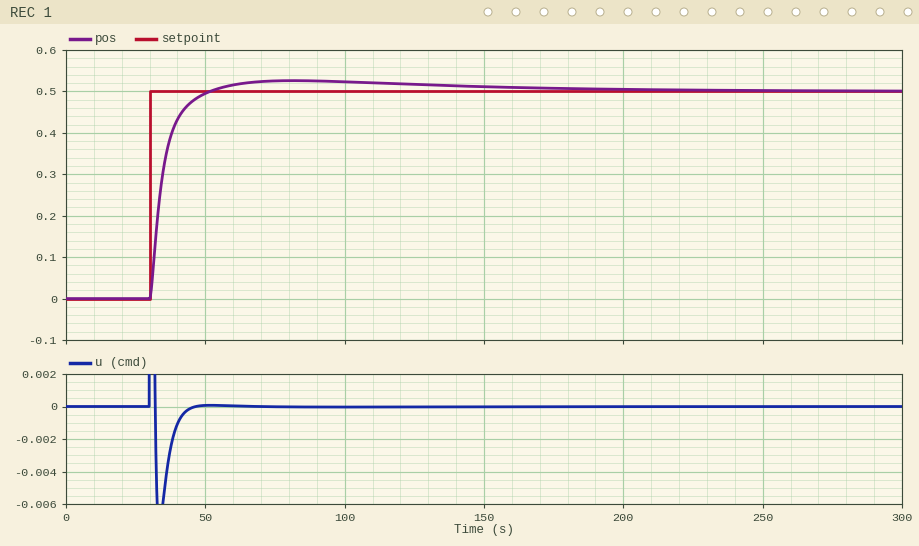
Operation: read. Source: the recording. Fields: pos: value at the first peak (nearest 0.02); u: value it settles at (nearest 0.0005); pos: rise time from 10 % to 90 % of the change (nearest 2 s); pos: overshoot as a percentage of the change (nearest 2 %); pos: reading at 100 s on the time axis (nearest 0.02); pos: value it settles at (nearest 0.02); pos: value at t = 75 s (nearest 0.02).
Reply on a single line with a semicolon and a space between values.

0.52; 0.0000; 10 s; 6 %; 0.52; 0.50; 0.52
